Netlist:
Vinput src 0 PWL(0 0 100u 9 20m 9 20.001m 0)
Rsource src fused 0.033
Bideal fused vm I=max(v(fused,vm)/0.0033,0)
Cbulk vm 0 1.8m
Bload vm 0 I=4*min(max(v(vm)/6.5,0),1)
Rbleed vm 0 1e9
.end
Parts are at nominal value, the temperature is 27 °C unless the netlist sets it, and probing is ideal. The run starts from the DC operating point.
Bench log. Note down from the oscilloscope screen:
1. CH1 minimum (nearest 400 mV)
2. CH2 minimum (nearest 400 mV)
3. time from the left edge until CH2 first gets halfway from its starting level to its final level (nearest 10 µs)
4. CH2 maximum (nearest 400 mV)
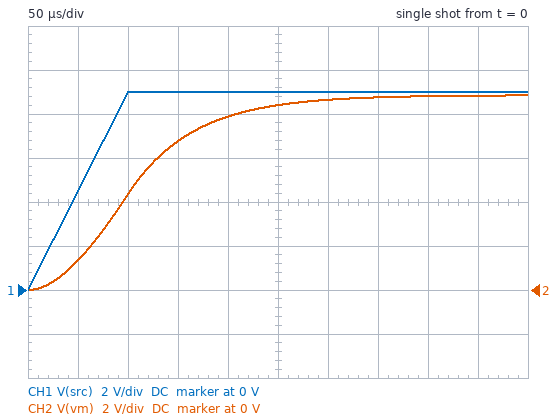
0 V
0 V
100 µs
8.8 V
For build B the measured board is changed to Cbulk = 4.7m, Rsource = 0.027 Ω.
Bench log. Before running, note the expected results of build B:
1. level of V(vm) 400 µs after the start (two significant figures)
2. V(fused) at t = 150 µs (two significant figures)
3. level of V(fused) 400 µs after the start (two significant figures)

8.1 V
4.9 V
8.2 V
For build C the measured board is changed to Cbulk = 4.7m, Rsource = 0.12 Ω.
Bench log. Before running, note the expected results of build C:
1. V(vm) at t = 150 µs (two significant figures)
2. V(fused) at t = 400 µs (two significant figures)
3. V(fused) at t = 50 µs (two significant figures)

1.4 V
4.1 V
300 mV
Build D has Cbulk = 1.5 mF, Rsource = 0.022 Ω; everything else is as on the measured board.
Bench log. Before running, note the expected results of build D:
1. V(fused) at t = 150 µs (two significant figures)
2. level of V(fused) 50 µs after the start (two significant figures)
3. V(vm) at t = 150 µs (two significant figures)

8.2 V
2.3 V
8.1 V
